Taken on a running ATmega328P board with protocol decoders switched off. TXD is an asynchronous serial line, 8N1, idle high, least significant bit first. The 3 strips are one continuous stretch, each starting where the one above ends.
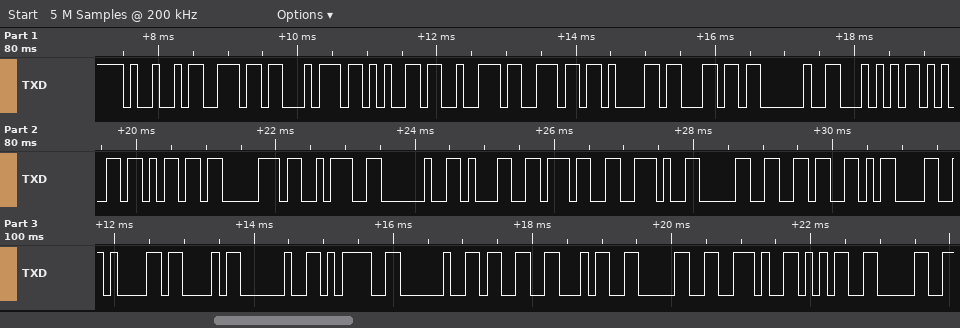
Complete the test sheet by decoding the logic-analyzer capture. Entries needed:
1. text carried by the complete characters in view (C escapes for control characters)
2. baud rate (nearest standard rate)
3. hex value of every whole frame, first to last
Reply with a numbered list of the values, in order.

1. "Internal Temp: 17.06\r\nC = 340.50"
2. 9600 baud
3. 49 6E 74 65 72 6E 61 6C 20 54 65 6D 70 3A 20 31 37 2E 30 36 0D 0A 43 20 3D 20 33 34 30 2E 35 30
